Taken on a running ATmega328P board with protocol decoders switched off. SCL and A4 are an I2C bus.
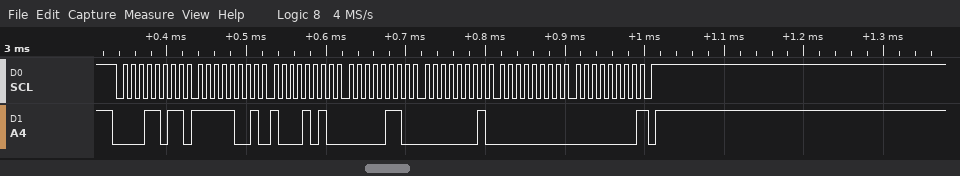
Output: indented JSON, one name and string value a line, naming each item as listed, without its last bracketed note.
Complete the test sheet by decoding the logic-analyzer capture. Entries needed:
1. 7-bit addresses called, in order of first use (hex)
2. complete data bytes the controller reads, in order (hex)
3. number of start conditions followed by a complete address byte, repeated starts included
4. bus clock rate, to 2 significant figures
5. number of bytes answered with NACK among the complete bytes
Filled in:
{
  "7-bit addresses called, in order of first use": "0x0D",
  "complete data bytes the controller reads, in order": "F9 8A 06 01 00 00",
  "number of start conditions followed by a complete address byte, repeated starts included": "1",
  "bus clock rate, to 2 significant figures": "100 kHz",
  "number of bytes answered with NACK among the complete bytes": "1"
}
